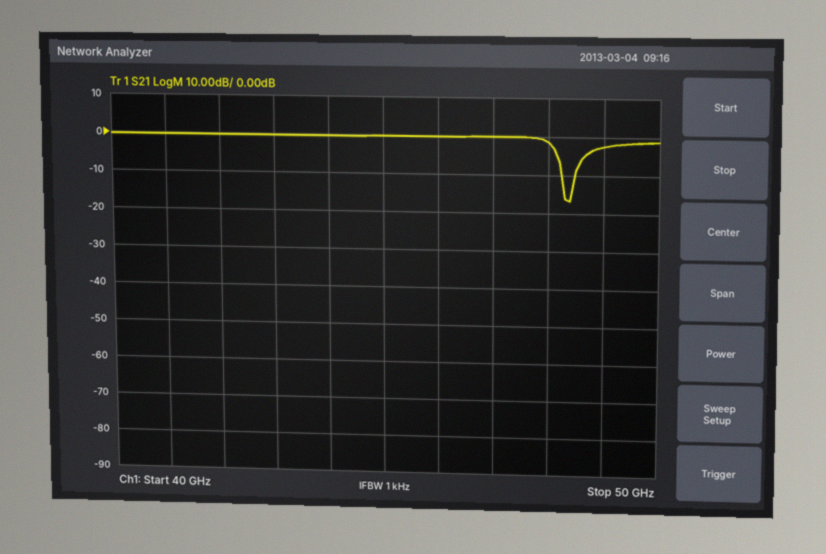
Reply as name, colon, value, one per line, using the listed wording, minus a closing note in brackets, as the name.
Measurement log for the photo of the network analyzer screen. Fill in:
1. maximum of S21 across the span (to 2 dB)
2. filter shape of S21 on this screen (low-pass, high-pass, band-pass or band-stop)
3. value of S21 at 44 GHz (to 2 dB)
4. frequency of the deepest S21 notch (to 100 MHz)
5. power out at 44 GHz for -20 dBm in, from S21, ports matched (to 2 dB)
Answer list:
maximum of S21 across the span: 0 dB
filter shape of S21 on this screen: band-stop
value of S21 at 44 GHz: 0 dB
frequency of the deepest S21 notch: 48.4 GHz
power out at 44 GHz for -20 dBm in, from S21, ports matched: -20 dBm
